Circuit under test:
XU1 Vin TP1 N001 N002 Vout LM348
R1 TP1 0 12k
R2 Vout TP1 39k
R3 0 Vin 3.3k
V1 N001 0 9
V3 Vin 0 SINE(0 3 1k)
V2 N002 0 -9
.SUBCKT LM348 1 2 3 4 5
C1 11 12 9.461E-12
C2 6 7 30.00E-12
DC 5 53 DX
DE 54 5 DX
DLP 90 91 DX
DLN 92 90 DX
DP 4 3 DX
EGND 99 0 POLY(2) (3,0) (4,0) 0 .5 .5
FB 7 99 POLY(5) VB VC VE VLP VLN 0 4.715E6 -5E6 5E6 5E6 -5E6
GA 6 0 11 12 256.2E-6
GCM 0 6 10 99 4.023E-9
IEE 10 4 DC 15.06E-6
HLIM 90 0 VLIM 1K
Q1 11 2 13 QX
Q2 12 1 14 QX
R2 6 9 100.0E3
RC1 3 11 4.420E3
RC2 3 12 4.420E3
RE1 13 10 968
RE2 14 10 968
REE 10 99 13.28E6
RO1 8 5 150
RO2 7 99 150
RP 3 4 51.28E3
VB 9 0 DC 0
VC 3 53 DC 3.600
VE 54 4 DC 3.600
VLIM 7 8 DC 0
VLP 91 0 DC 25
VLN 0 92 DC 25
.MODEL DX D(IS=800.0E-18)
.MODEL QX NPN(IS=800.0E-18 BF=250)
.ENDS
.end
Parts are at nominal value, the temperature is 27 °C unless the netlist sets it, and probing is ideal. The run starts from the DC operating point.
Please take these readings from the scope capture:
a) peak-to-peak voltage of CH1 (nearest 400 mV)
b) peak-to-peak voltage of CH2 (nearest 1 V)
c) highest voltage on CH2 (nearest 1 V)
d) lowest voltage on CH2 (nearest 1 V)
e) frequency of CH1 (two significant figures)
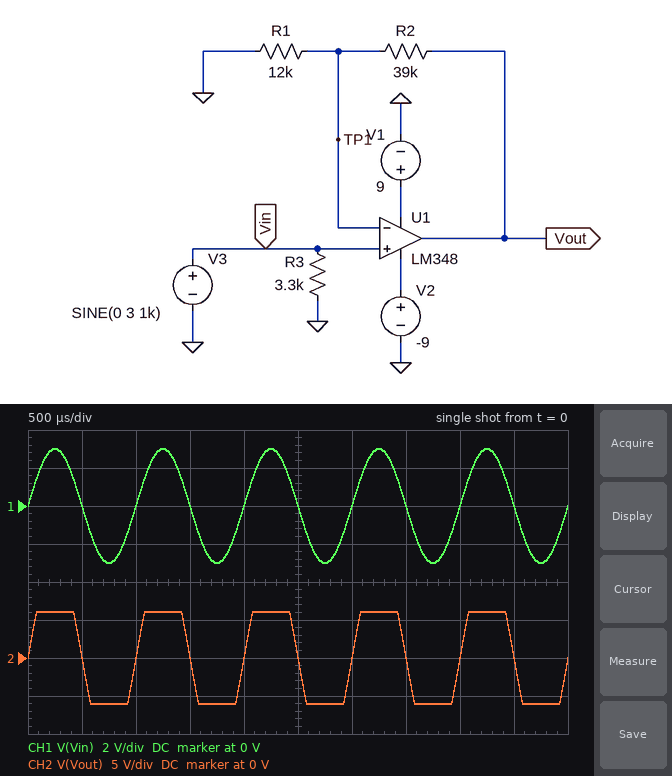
6.0 V
12 V
6 V
-6 V
1.0 kHz
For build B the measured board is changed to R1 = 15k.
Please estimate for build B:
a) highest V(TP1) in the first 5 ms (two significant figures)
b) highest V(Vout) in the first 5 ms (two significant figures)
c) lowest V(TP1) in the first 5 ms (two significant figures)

1.7 V
6.0 V
-1.7 V
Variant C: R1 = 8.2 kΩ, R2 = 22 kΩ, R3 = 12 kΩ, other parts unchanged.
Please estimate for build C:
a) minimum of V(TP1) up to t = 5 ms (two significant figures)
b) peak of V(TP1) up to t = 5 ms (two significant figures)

-1.6 V
1.6 V
